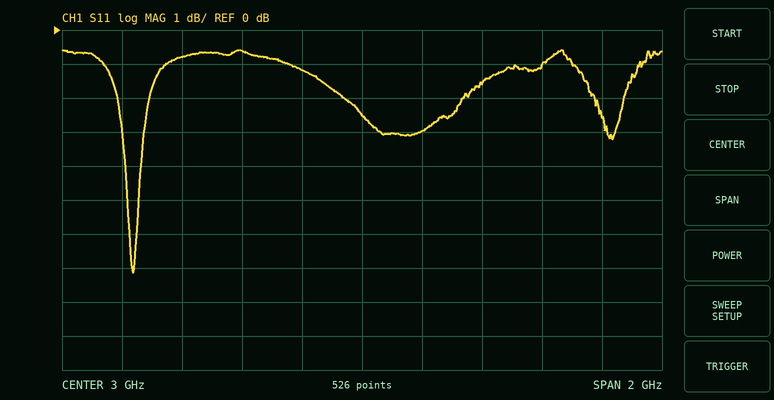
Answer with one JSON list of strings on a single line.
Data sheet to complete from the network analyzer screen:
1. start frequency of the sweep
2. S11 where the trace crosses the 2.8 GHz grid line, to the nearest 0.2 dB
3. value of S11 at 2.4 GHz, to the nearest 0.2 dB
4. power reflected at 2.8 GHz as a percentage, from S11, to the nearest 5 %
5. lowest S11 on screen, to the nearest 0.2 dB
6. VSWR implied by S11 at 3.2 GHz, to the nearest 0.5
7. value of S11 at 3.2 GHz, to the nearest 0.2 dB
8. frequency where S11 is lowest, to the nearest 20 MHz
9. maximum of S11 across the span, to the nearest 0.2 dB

["2 GHz", "-1.2 dB", "-0.8 dB", "75 %", "-7.2 dB", "6.0", "-3.0 dB", "2.24 GHz", "-0.6 dB"]
